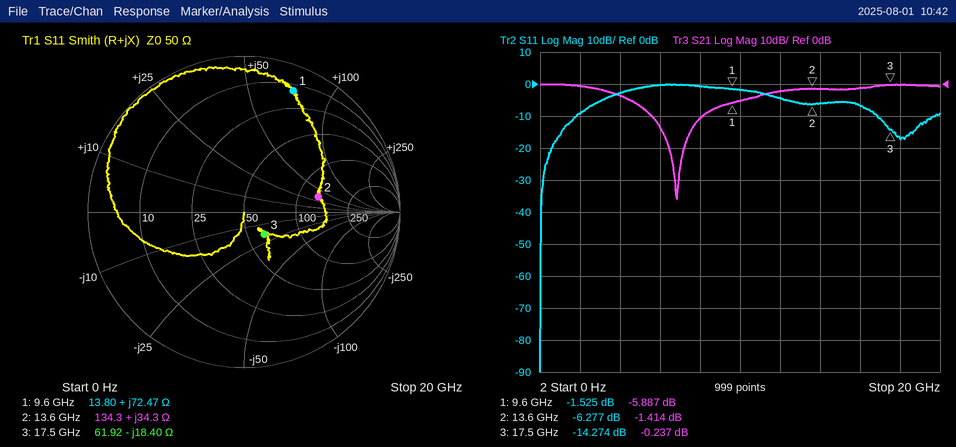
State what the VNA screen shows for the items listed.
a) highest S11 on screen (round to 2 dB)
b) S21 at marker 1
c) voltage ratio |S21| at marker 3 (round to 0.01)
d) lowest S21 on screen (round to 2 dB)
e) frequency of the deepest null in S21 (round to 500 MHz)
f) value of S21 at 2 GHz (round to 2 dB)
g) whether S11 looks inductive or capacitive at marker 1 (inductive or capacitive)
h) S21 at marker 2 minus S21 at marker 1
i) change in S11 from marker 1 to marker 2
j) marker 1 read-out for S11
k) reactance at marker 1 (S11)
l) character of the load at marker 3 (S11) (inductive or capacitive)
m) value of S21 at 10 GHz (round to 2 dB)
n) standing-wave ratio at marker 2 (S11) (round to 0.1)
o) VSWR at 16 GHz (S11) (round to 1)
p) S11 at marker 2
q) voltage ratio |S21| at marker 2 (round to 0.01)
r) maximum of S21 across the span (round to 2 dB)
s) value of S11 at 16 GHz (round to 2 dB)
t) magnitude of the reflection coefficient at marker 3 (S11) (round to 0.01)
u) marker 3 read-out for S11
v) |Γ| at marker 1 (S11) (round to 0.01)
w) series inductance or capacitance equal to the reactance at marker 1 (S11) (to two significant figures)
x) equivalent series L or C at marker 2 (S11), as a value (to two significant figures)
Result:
0 dB
-5.887 dB
0.97
-36 dB
7.0 GHz
0 dB
inductive
4.473 dB
-4.752 dB
-1.525 dB
+72.47 Ω
capacitive
-6 dB
2.9
3
-6.277 dB
0.85
0 dB
-6 dB
0.19
-14.274 dB
0.84
1.2 nH
400 pH
